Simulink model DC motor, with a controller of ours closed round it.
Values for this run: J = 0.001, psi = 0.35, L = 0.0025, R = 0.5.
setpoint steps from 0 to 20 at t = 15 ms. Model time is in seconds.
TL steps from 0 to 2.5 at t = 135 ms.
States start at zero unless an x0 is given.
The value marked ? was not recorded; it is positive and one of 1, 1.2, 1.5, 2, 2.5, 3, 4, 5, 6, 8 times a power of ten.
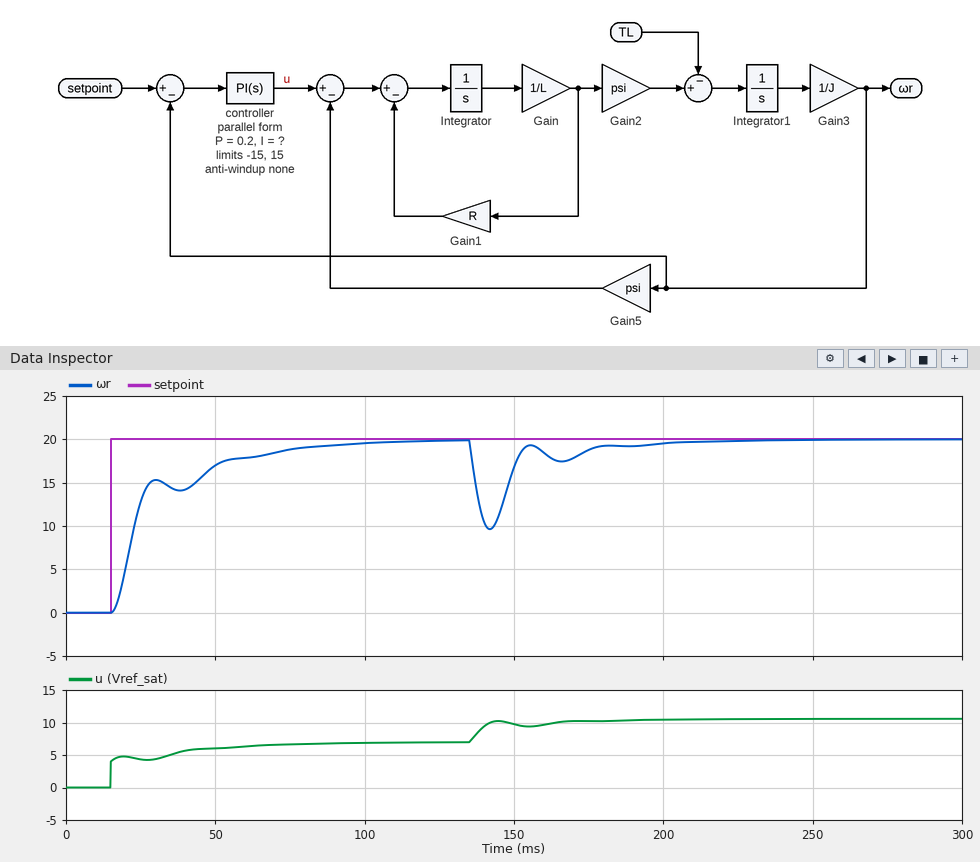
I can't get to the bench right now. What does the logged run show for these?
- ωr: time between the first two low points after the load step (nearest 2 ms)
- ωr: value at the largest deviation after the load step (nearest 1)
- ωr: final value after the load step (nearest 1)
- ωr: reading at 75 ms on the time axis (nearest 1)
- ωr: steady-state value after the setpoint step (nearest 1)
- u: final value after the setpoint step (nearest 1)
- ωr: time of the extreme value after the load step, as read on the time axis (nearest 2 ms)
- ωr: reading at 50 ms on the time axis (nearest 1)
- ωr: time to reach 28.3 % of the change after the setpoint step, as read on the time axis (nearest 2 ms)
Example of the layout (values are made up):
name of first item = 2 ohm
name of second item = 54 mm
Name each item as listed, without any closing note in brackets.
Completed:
ωr: time between the first two low points after the load step = 24 ms
ωr: value at the largest deviation after the load step = 10
ωr: final value after the load step = 20
ωr: reading at 75 ms on the time axis = 19
ωr: steady-state value after the setpoint step = 20
u: final value after the setpoint step = 7
ωr: time of the extreme value after the load step, as read on the time axis = 142 ms
ωr: reading at 50 ms on the time axis = 17
ωr: time to reach 28.3 % of the change after the setpoint step, as read on the time axis = 20 ms
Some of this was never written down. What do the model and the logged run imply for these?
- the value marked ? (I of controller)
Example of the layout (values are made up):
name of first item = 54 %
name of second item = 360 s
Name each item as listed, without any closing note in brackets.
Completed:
the value marked ? = 20
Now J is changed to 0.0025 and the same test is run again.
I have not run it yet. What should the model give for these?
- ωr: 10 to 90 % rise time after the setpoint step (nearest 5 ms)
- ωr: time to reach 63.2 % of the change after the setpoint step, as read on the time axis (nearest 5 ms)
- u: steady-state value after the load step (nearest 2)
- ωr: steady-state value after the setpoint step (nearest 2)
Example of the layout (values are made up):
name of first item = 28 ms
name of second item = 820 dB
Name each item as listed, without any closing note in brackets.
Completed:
ωr: 10 to 90 % rise time after the setpoint step = 25 ms
ωr: time to reach 63.2 % of the change after the setpoint step, as read on the time axis = 30 ms
u: steady-state value after the load step = 10
ωr: steady-state value after the setpoint step = 20
